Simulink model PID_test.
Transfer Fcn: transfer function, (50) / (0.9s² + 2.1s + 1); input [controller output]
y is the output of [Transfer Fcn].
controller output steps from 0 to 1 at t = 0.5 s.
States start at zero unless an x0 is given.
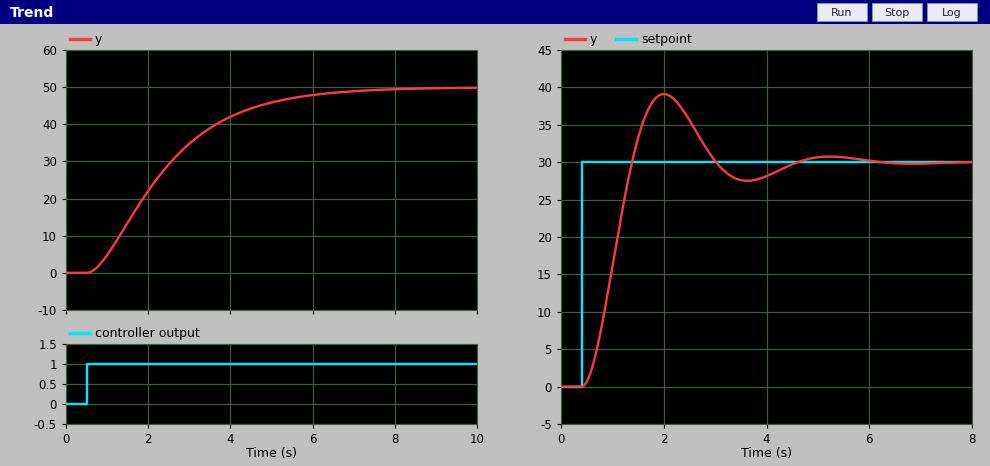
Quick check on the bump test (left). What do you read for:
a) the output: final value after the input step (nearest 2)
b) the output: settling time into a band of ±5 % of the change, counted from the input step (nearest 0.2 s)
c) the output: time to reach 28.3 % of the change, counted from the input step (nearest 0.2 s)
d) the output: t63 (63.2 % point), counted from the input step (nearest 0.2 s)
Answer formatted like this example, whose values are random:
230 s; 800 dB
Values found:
50; 5.2 s; 1.0 s; 2.2 s
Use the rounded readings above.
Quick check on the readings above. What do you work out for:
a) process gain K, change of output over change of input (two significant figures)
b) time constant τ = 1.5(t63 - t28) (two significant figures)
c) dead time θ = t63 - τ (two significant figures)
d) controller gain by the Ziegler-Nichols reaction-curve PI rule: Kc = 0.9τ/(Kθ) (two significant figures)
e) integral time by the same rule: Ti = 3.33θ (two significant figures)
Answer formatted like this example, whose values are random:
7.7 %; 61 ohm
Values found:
50; 1.8 s; 0.40 s; 0.081; 1.3 s
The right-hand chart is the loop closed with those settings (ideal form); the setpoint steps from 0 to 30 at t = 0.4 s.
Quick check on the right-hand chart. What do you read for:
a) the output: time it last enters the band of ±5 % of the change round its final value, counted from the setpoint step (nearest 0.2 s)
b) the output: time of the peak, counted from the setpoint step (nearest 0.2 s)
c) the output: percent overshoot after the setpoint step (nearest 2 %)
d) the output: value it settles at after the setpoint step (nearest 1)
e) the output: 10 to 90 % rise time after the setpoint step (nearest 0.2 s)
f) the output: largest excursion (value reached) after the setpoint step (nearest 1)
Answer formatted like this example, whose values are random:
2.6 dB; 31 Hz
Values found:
3.8 s; 1.6 s; 30 %; 30; 0.6 s; 39
